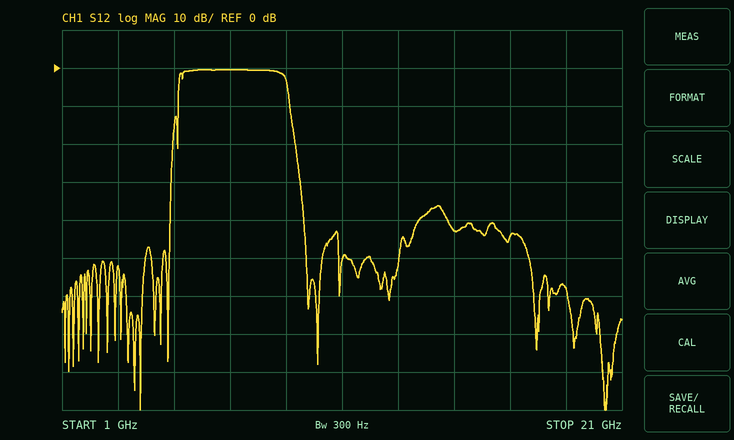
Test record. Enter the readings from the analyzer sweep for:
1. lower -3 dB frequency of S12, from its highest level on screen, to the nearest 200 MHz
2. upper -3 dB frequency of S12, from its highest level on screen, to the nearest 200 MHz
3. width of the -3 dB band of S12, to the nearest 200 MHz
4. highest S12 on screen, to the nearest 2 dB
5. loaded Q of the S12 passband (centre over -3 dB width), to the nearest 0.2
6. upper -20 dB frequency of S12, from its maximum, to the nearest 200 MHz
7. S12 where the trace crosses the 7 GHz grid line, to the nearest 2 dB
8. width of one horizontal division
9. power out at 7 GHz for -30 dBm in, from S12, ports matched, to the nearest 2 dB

5.2 GHz
9.0 GHz
3.8 GHz
0 dB
1.8
9.4 GHz
0 dB
2 GHz
-30 dBm
